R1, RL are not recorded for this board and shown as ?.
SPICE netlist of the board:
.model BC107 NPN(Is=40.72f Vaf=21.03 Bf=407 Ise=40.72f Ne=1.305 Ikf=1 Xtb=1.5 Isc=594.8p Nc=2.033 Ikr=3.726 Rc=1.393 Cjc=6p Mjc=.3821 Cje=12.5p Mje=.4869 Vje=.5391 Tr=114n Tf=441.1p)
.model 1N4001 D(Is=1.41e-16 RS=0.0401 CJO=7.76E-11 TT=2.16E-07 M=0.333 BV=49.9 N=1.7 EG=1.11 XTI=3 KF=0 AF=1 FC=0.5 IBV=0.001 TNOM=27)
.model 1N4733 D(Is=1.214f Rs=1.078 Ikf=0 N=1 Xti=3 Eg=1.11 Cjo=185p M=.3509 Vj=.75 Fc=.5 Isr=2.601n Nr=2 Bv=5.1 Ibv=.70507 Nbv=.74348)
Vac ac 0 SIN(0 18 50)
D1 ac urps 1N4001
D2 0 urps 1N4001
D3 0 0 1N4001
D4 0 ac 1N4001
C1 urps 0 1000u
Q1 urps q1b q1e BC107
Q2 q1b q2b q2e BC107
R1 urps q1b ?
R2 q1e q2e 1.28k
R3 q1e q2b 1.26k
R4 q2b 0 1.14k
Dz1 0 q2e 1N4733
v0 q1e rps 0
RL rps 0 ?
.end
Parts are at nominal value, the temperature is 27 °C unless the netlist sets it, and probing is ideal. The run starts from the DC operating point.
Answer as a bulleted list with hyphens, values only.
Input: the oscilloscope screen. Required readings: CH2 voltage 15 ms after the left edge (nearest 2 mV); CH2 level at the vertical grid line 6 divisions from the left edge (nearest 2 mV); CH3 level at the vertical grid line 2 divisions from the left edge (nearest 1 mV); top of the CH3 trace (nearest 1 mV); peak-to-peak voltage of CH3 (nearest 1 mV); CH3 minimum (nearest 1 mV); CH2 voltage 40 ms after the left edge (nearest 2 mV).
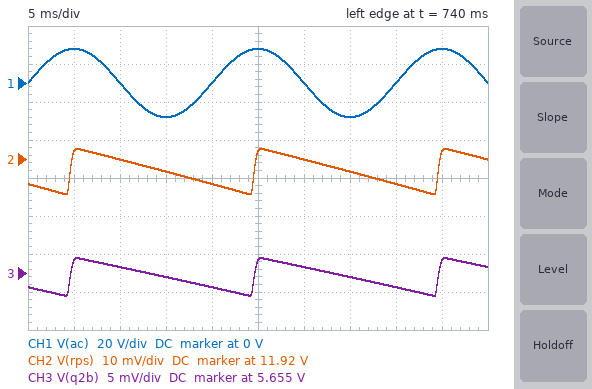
- 11.916 V
- 11.920 V
- 5.656 V
- 5.657 V
- 5 mV
- 5.652 V
- 11.914 V
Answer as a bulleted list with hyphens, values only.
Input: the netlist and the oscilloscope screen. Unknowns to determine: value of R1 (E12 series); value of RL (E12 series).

- 1.5 kΩ
- 820 Ω
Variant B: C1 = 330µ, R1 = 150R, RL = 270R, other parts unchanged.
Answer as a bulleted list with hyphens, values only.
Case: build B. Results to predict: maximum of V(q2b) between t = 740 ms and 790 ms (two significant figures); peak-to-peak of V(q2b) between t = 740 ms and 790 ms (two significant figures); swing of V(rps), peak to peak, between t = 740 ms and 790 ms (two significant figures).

- 5.8 V
- 120 mV
- 340 mV
